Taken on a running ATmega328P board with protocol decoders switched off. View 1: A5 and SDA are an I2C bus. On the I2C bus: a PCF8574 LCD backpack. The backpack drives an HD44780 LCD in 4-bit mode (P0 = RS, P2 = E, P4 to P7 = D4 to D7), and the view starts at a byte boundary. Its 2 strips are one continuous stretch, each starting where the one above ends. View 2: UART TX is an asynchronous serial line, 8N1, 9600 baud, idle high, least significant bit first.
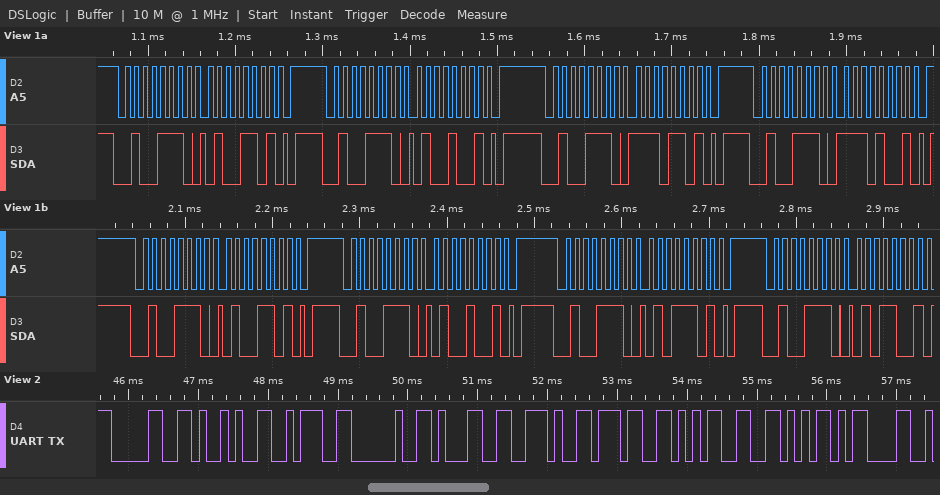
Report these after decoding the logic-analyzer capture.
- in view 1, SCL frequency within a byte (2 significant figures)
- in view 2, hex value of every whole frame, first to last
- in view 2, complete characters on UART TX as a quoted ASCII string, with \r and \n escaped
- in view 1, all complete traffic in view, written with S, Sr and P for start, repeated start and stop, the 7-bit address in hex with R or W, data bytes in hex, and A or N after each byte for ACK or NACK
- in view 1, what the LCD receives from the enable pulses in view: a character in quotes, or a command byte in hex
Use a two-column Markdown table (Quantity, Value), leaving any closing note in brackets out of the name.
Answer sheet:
| Quantity | Value |
|---|---|
| in view 1, SCL frequency within a byte | 100 kHz |
| in view 2, hex value of every whole frame, first to last | 0x30 0x29 0x3A 0x20 0x31 0x2E 0x37 0x35 0x56 0x0D |
| in view 2, complete characters on UART TX as a quoted ASCII string, with \r and \n escaped | "0): 1.75V\r" |
| in view 1, all complete traffic in view, written with S, Sr and P for start, repeated start and stop, the 7-bit address in hex with R or W, data bytes in hex, and A or N after each byte for ACK or NACK | S 27W A 4D A P S 27W A 49 A P S 27W A ED A P S 27W A E9 A P S 27W A 4D A P S 27W A 49 A P S 27W A 5D A P S 27W A 59 A |
| in view 1, what the LCD receives from the enable pulses in view: a character in quotes, or a command byte in hex | 'N' 'E' |
